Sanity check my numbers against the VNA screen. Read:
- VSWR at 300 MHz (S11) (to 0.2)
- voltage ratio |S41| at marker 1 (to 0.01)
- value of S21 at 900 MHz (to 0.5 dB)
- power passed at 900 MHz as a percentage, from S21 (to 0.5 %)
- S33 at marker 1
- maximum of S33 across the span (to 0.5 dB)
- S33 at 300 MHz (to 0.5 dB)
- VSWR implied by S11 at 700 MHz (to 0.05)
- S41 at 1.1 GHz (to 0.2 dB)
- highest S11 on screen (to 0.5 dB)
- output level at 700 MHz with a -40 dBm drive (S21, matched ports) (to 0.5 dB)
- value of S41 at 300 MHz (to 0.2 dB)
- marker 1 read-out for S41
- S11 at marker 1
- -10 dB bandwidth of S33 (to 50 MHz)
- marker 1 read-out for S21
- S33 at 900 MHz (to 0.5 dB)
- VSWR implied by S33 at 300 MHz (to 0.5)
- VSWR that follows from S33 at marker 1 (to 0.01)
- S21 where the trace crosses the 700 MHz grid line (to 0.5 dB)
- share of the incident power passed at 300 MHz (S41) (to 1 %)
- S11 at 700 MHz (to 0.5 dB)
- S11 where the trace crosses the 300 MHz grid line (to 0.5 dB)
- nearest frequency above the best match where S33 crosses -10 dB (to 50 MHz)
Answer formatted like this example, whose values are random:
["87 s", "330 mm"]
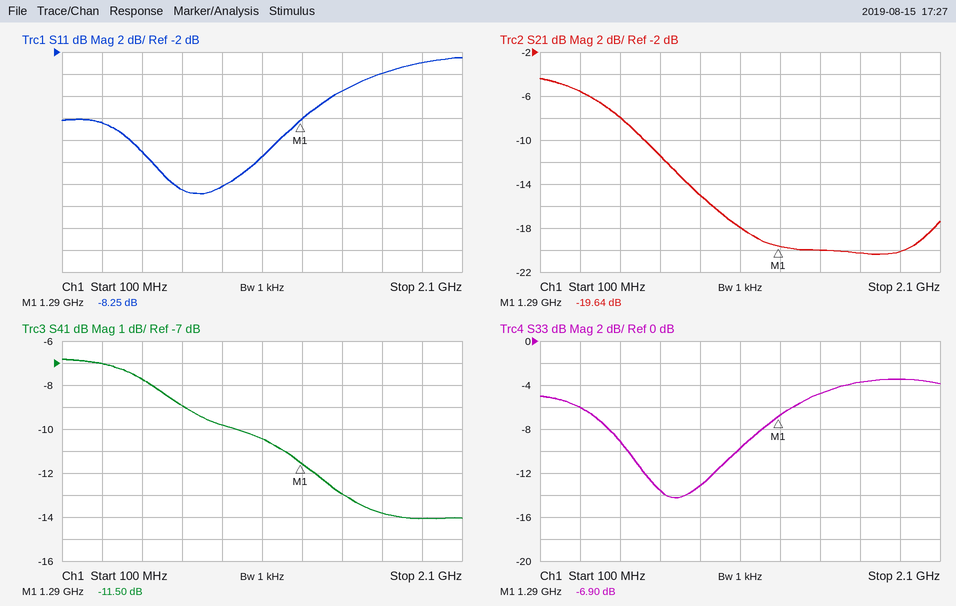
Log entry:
["2.2", "0.27", "-15.0 dB", "3.0 %", "-6.90 dB", "-3.5 dB", "-6.0 dB", "1.45", "-10.4 dB", "-2.5 dB", "-51.5 dBm", "-7.0 dB", "-11.50 dB", "-8.25 dB", "550 MHz", "-19.64 dB", "-13.0 dB", "3.0", "2.65", "-11.5 dB", "20 %", "-14.5 dB", "-8.5 dB", "1.10 GHz"]
